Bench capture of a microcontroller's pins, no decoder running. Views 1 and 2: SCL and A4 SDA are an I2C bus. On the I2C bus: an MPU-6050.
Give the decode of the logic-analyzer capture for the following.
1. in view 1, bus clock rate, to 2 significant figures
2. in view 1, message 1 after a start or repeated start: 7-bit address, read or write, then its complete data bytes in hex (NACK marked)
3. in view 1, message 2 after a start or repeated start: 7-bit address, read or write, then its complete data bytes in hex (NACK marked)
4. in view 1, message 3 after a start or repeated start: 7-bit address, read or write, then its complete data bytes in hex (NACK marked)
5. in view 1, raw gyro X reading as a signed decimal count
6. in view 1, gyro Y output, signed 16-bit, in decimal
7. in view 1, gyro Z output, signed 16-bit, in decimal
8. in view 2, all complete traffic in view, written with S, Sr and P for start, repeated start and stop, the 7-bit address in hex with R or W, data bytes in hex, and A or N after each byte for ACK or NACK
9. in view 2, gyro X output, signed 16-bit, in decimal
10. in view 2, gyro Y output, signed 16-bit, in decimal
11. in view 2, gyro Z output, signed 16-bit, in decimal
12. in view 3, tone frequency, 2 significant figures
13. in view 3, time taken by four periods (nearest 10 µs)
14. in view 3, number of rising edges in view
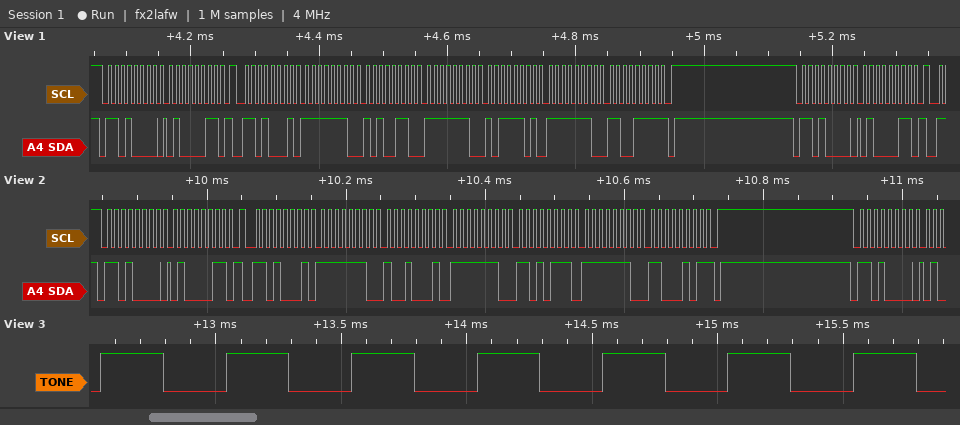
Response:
100 kHz
0x68 write: 43
0x68 read: FE A6 FE BD FE CF NACK
0x68 write: 43
-346
-323
-305
S 68W A 43 A Sr 68R A FE A 91 A FE A D7 A FE A C5 N P S 68W A
-367
-297
-315
2.0 kHz
2000 µs
7
